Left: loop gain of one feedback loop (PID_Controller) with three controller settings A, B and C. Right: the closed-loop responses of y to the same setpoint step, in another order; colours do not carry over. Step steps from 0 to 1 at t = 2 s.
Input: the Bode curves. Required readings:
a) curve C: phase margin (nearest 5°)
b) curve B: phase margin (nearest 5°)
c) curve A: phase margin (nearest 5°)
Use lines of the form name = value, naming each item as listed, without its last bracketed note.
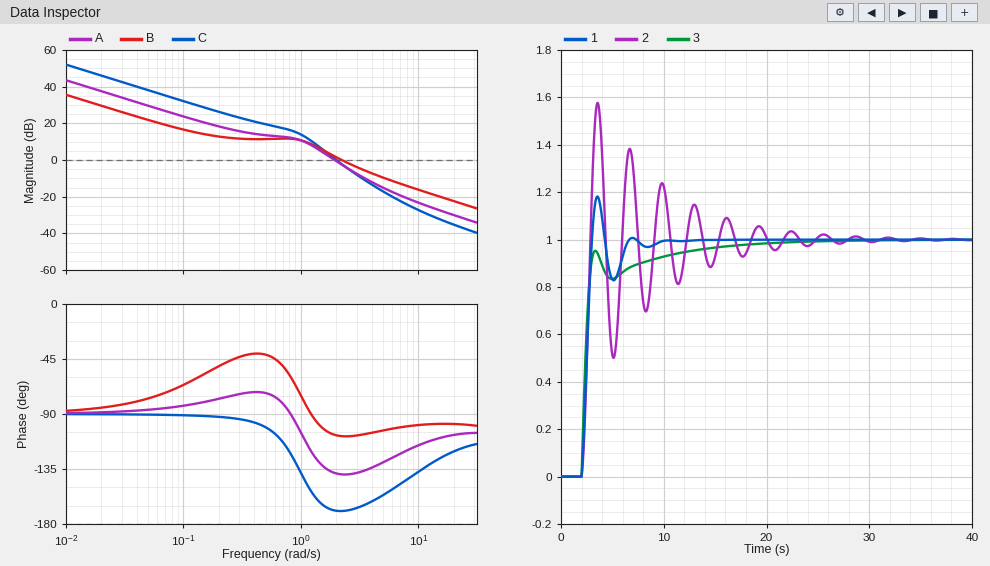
curve C: phase margin = 10°
curve B: phase margin = 70°
curve A: phase margin = 40°
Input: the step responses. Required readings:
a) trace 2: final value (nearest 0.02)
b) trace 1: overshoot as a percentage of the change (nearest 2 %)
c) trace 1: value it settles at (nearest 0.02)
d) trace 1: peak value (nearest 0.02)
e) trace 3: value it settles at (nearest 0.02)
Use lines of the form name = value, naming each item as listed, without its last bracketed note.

trace 2: final value = 1.00
trace 1: overshoot as a percentage of the change = 18 %
trace 1: value it settles at = 1.00
trace 1: peak value = 1.18
trace 3: value it settles at = 1.00
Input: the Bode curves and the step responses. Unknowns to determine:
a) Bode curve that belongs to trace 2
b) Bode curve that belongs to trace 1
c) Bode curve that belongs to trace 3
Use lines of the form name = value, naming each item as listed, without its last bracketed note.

Bode curve that belongs to trace 2 = C
Bode curve that belongs to trace 1 = A
Bode curve that belongs to trace 3 = B
